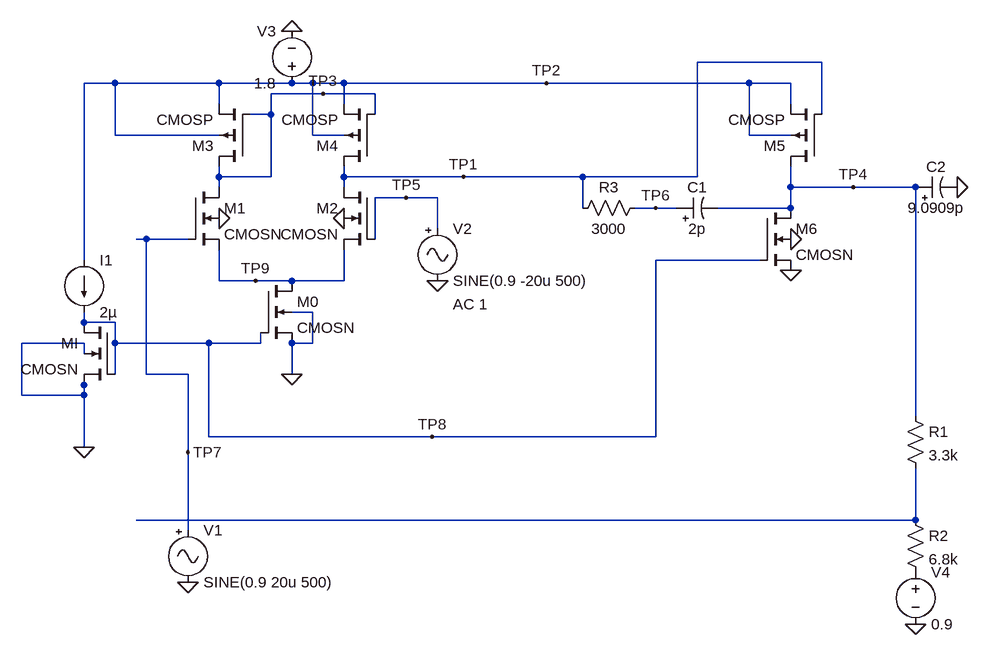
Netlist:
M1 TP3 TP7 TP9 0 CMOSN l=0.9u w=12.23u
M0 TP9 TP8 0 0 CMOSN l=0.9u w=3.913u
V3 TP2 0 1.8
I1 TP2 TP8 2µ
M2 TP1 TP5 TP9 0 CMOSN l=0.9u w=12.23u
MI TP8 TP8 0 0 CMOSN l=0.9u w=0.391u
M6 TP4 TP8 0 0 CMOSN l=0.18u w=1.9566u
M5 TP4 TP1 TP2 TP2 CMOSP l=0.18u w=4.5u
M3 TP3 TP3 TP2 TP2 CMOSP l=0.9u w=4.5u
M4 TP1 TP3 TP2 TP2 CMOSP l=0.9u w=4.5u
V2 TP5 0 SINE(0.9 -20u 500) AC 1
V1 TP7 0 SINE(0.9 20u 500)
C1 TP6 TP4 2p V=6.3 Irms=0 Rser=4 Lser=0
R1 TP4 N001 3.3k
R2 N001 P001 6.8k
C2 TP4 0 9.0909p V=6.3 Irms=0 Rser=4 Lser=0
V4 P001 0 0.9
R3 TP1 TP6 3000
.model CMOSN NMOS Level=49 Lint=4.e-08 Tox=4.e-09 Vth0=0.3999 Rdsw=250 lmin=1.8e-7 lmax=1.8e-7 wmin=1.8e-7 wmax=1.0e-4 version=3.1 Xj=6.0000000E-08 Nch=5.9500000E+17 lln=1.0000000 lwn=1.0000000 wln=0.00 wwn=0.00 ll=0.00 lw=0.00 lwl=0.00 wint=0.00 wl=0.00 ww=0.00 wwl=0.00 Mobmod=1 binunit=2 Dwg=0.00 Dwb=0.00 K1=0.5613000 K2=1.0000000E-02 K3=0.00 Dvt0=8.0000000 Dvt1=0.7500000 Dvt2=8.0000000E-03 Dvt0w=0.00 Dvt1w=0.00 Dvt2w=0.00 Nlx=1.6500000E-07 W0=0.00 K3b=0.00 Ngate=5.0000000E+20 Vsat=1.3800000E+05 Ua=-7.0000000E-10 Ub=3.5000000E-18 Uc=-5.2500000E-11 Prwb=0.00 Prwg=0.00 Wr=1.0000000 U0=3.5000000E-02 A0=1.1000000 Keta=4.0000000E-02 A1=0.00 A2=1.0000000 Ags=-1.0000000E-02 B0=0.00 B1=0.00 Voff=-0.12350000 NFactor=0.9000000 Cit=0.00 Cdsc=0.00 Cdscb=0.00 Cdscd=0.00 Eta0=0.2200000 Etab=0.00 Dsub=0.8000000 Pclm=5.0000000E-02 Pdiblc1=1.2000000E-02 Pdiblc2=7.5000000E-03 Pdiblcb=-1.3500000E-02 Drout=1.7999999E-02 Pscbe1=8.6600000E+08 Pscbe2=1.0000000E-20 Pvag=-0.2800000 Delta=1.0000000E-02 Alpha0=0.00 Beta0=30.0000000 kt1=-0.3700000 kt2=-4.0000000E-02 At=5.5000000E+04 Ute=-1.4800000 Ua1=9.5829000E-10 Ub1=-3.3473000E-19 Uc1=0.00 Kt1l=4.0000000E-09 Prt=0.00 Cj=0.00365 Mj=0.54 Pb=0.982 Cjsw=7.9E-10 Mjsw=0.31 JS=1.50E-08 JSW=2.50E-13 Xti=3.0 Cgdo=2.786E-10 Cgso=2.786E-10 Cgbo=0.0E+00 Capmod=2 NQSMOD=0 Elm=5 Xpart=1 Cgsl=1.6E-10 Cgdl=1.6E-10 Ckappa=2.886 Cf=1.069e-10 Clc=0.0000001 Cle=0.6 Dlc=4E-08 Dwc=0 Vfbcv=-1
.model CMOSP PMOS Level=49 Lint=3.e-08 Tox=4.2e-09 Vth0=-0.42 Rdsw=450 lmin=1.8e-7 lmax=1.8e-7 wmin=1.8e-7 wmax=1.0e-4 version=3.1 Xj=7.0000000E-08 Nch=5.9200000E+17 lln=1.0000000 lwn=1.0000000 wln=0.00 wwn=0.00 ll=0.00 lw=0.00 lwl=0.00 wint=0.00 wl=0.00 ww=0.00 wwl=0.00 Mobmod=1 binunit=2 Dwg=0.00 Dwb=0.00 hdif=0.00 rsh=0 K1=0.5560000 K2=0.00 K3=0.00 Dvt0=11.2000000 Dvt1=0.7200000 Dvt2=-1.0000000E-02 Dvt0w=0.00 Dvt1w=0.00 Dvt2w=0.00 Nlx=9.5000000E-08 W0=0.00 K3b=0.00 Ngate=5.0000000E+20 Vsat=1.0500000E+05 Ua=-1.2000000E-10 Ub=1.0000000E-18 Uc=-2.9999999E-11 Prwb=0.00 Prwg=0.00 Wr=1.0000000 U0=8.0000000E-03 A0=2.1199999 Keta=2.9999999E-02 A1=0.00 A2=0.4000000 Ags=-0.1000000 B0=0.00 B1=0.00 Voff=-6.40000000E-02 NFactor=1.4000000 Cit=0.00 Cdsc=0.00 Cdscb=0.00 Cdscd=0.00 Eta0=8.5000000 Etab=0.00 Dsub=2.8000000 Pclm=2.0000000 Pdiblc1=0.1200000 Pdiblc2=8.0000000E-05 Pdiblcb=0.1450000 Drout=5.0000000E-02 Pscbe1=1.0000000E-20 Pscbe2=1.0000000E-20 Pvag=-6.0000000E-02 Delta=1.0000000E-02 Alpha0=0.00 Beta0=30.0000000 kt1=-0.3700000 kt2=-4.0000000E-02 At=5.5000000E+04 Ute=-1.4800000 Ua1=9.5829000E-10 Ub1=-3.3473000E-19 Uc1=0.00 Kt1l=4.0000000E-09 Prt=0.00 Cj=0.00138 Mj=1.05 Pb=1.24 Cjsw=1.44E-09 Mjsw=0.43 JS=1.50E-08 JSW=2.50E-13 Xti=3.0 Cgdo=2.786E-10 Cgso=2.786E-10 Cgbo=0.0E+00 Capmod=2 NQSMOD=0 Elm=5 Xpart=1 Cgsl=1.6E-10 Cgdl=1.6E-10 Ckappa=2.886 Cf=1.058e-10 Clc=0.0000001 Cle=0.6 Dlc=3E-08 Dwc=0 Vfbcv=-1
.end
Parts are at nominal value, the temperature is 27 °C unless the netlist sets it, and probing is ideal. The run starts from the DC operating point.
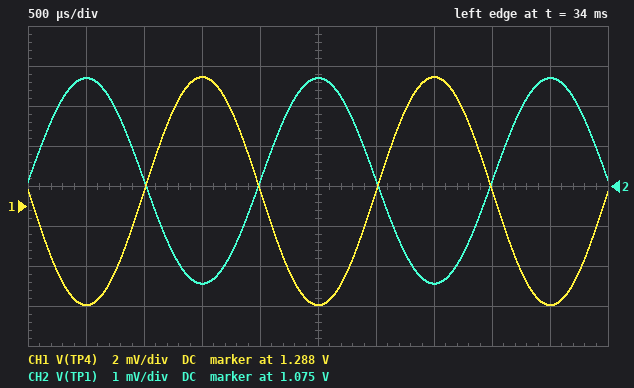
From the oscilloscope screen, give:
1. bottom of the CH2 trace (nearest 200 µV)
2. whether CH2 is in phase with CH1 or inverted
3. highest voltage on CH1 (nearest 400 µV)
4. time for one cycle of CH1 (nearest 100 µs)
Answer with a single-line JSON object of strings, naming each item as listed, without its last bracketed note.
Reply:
{"bottom of the CH2 trace": "1.0726 V", "whether CH2 is in phase with CH1 or inverted": "inverted", "highest voltage on CH1": "1.2944 V", "time for one cycle of CH1": "2.0 ms"}
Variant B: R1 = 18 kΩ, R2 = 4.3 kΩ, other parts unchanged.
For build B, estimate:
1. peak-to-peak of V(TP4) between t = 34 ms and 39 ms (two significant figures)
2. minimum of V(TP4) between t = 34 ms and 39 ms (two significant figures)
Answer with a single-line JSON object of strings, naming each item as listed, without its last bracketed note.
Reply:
{"peak-to-peak of V(TP4) between t = 34 ms and 39 ms": "12 mV", "minimum of V(TP4) between t = 34 ms and 39 ms": "1.4 V"}
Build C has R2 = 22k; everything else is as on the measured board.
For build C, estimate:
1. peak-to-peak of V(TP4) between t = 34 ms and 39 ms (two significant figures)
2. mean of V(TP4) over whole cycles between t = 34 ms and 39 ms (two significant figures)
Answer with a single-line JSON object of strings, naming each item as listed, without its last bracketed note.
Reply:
{"peak-to-peak of V(TP4) between t = 34 ms and 39 ms": "12 mV", "mean of V(TP4) over whole cycles between t = 34 ms and 39 ms": "1.4 V"}
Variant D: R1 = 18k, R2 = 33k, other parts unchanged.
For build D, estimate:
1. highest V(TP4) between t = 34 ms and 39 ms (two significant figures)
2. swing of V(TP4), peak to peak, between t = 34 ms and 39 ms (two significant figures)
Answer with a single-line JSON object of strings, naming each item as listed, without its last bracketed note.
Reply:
{"highest V(TP4) between t = 34 ms and 39 ms": "1.4 V", "swing of V(TP4), peak to peak, between t = 34 ms and 39 ms": "12 mV"}
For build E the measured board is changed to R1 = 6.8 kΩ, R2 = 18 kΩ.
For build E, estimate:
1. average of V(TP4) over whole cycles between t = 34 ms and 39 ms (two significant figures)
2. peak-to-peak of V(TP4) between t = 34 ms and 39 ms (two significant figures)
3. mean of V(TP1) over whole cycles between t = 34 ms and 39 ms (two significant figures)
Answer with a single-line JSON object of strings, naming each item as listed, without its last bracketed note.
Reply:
{"average of V(TP4) over whole cycles between t = 34 ms and 39 ms": "1.4 V", "peak-to-peak of V(TP4) between t = 34 ms and 39 ms": "12 mV", "mean of V(TP1) over whole cycles between t = 34 ms and 39 ms": "1.1 V"}
